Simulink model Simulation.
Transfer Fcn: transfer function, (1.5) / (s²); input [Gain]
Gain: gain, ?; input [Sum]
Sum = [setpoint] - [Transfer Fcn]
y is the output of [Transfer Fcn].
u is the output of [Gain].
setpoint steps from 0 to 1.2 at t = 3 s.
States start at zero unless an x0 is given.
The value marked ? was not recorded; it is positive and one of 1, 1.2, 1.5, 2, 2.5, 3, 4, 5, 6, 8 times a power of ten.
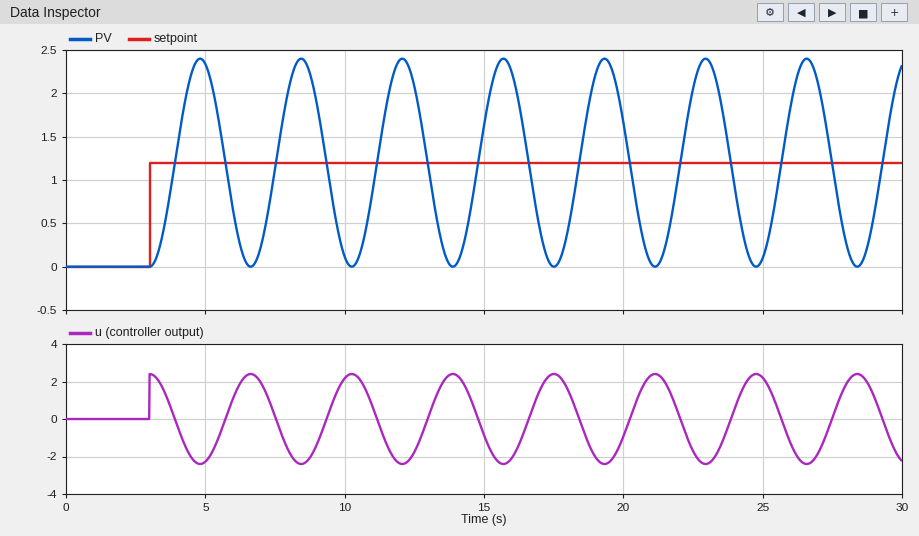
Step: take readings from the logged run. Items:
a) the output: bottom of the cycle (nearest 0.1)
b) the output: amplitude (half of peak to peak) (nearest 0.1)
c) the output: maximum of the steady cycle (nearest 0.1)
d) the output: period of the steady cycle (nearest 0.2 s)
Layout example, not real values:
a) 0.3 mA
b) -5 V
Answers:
a) 0.0
b) 1.2
c) 2.4
d) 3.6 s
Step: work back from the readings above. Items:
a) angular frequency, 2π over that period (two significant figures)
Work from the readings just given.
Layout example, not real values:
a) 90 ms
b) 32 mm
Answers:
a) 1.7 rad/s
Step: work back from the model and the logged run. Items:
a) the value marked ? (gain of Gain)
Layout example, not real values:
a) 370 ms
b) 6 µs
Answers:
a) 2
